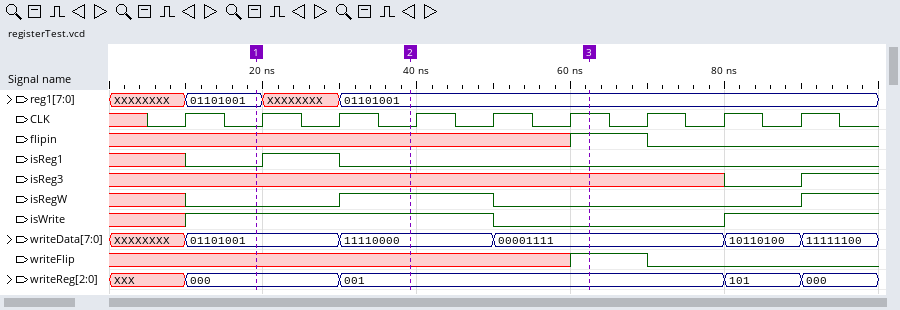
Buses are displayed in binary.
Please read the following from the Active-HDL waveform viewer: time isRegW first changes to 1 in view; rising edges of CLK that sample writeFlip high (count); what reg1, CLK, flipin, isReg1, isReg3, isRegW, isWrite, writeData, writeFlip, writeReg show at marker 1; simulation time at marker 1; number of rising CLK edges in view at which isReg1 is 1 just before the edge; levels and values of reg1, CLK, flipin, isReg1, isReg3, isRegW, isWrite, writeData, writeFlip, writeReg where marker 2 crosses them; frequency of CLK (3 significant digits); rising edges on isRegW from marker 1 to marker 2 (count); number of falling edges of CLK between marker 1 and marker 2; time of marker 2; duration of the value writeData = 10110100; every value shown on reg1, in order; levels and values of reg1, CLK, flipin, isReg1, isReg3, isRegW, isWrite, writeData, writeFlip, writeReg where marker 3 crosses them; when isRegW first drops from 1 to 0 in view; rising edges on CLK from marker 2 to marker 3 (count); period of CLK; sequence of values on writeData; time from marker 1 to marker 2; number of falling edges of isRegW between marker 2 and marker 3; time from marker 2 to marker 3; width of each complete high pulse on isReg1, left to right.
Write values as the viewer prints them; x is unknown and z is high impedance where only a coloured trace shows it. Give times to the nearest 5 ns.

30 ns
1
reg1=01101001, CLK=0, flipin=x, isReg1=0, isReg3=x, isRegW=0, isWrite=1, writeData=01101001, writeFlip=x, writeReg=000
20 ns
1
reg1=01101001, CLK=0, flipin=x, isReg1=0, isReg3=x, isRegW=1, isWrite=1, writeData=11110000, writeFlip=x, writeReg=001
100 MHz
1
2
40 ns
10 ns
XXXXXXXX, 01101001, XXXXXXXX, 01101001
reg1=01101001, CLK=1, flipin=1, isReg1=0, isReg3=x, isRegW=0, isWrite=0, writeData=00001111, writeFlip=1, writeReg=001
50 ns
3
10 ns
XXXXXXXX, 01101001, 11110000, 00001111, 10110100, 11111100
20 ns
1
25 ns
10 ns
